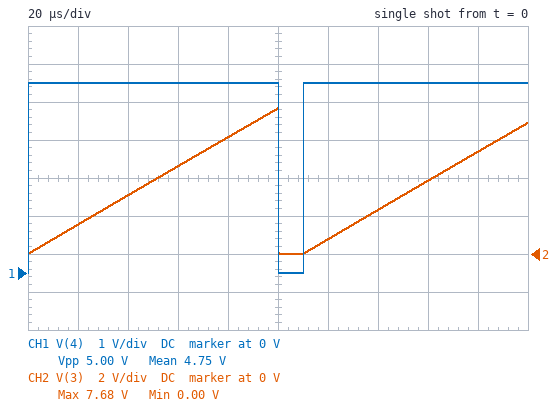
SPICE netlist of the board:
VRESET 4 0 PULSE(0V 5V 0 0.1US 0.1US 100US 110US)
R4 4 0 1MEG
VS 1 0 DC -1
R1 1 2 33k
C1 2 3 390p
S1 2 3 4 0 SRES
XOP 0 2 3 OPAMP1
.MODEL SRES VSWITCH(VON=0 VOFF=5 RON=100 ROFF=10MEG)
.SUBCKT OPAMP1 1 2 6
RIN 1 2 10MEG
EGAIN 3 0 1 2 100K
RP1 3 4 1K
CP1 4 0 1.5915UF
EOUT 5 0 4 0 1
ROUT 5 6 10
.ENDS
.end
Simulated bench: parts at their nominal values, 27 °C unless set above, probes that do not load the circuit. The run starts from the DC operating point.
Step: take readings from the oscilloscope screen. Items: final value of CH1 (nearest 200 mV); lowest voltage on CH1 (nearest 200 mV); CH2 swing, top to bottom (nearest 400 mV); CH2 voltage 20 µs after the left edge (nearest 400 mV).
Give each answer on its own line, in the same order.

5.0 V
0 V
7.6 V
1.6 V
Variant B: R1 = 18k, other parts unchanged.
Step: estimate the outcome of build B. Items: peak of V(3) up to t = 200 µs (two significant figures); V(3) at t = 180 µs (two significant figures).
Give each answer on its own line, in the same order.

14 V
9.9 V
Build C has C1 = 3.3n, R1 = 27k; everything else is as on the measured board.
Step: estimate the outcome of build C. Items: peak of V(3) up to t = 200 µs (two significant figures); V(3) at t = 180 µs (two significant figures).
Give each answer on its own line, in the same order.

1.1 V
790 mV
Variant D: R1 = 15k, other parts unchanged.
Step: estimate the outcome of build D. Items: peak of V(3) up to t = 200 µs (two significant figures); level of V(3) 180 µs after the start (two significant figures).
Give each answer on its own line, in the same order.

17 V
12 V
